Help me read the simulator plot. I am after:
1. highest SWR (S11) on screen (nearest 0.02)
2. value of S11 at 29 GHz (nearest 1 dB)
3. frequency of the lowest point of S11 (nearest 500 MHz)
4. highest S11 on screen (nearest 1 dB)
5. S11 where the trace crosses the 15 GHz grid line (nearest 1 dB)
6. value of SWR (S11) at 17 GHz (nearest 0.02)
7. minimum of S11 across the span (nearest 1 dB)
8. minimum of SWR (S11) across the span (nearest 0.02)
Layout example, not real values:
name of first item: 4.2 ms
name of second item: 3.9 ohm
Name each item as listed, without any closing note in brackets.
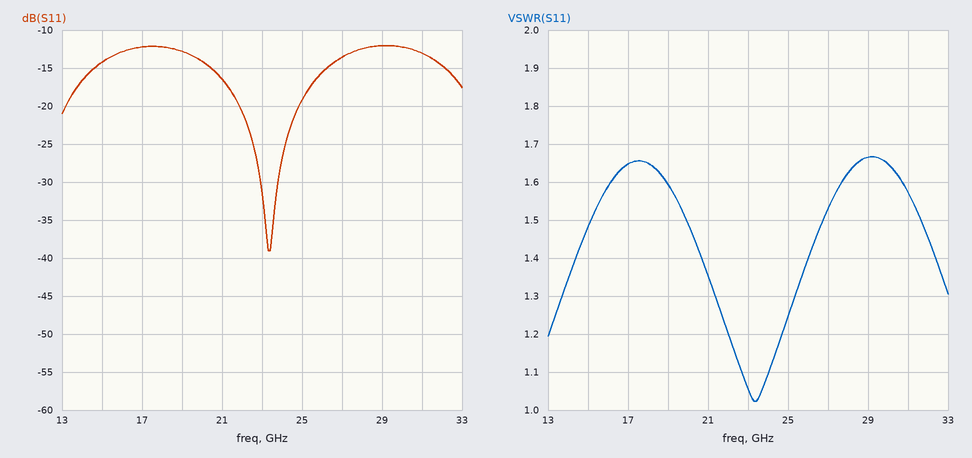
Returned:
highest SWR (S11) on screen: 1.66
value of S11 at 29 GHz: -12 dB
frequency of the lowest point of S11: 23.5 GHz
highest S11 on screen: -12 dB
S11 where the trace crosses the 15 GHz grid line: -14 dB
value of SWR (S11) at 17 GHz: 1.64
minimum of S11 across the span: -39 dB
minimum of SWR (S11) across the span: 1.02
